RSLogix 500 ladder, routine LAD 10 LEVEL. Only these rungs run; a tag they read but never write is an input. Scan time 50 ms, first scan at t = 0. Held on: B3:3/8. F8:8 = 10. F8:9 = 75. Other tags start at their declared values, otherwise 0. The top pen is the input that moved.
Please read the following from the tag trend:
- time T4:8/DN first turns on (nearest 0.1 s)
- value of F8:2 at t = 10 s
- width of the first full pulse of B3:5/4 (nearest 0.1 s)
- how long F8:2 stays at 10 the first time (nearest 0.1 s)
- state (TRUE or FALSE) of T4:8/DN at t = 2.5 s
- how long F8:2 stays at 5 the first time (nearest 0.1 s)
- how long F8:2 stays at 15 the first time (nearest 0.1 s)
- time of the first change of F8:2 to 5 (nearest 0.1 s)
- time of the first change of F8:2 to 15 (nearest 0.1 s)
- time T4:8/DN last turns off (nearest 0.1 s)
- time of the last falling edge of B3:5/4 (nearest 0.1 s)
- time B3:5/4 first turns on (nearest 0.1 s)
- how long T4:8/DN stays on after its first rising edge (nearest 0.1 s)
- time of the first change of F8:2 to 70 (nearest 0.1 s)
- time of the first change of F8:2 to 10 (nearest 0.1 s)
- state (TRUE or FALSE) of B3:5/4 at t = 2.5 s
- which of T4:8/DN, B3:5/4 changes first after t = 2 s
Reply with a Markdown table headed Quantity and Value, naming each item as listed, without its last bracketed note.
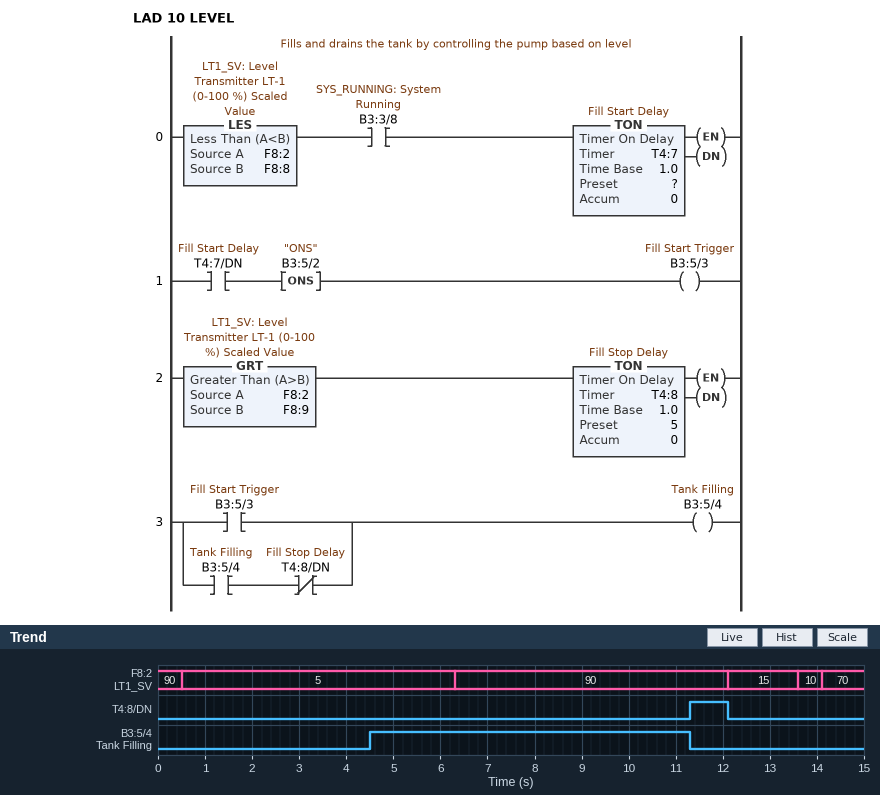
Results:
| Quantity | Value |
|---|---|
| time T4:8/DN first turns on | 11.3 s |
| value of F8:2 at t = 10 s | 90 |
| width of the first full pulse of B3:5/4 | 6.8 s |
| how long F8:2 stays at 10 the first time | 0.5 s |
| state (TRUE or FALSE) of T4:8/DN at t = 2.5 s | FALSE |
| how long F8:2 stays at 5 the first time | 5.8 s |
| how long F8:2 stays at 15 the first time | 1.5 s |
| time of the first change of F8:2 to 5 | 0.5 s |
| time of the first change of F8:2 to 15 | 12.1 s |
| time T4:8/DN last turns off | 12.1 s |
| time of the last falling edge of B3:5/4 | 11.3 s |
| time B3:5/4 first turns on | 4.5 s |
| how long T4:8/DN stays on after its first rising edge | 0.8 s |
| time of the first change of F8:2 to 70 | 14.1 s |
| time of the first change of F8:2 to 10 | 13.6 s |
| state (TRUE or FALSE) of B3:5/4 at t = 2.5 s | FALSE |
| which of T4:8/DN, B3:5/4 changes first after t = 2 s | B3:5/4 |
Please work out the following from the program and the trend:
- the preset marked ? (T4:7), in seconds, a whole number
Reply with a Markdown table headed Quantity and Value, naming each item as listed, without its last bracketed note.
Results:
| Quantity | Value |
|---|---|
| the preset marked ? (T4:7), in seconds, a whole number | 4 s |
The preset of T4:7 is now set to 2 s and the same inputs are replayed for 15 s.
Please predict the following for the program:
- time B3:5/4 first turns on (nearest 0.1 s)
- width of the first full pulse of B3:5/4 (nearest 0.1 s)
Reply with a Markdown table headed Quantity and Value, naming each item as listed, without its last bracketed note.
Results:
| Quantity | Value |
|---|---|
| time B3:5/4 first turns on | 2.5 s |
| width of the first full pulse of B3:5/4 | 8.8 s |
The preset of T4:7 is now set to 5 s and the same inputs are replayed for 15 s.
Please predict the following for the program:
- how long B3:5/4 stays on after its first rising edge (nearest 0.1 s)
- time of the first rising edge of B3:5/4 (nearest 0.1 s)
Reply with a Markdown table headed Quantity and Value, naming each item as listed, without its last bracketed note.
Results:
| Quantity | Value |
|---|---|
| how long B3:5/4 stays on after its first rising edge | 5.8 s |
| time of the first rising edge of B3:5/4 | 5.5 s |
